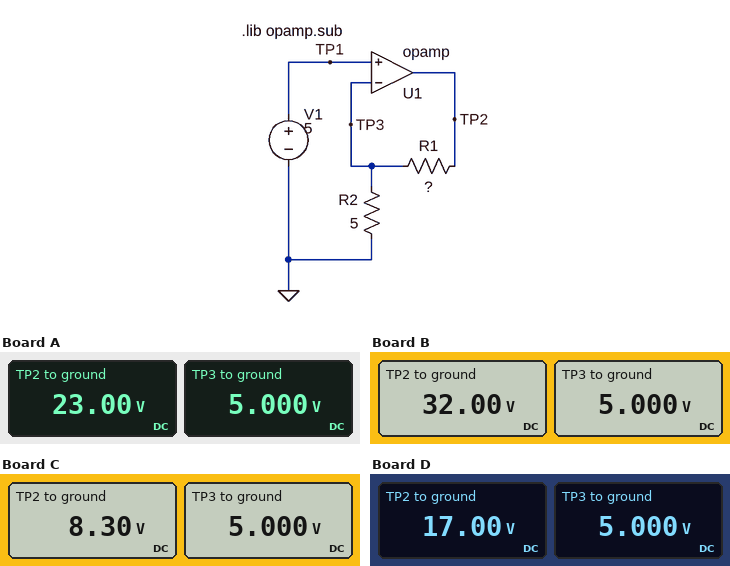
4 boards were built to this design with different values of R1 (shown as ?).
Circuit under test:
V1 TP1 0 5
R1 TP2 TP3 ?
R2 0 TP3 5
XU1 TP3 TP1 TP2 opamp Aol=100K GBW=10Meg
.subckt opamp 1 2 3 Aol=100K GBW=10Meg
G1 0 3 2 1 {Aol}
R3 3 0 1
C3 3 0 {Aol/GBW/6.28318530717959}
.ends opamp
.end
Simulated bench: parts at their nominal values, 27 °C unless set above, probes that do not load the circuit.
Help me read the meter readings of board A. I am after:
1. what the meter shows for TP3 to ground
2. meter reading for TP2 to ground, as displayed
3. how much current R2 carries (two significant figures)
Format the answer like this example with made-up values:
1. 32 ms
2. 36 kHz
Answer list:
1. 5.000 V
2. 23.00 V
3. 1.0 A
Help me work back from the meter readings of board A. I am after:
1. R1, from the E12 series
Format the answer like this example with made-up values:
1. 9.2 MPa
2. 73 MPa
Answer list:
1. 18 Ω
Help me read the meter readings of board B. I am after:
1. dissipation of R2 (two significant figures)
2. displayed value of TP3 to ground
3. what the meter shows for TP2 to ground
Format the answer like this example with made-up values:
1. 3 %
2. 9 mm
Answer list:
1. 5.0 W
2. 5.000 V
3. 32.00 V
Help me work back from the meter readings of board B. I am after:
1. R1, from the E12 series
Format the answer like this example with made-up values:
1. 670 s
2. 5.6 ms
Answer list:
1. 27 Ω
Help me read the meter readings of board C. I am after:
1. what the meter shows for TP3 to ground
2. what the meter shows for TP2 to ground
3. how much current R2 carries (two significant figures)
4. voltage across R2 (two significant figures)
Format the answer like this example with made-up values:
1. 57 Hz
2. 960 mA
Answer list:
1. 5.000 V
2. 8.30 V
3. 1.0 A
4. 5.0 V
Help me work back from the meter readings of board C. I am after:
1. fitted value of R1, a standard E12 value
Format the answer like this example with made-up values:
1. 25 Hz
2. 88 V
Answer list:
1. 3.3 Ω
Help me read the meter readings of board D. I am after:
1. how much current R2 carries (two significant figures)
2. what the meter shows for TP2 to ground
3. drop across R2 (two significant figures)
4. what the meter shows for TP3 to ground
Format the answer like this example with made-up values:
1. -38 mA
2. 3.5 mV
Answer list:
1. 1.0 A
2. 17.00 V
3. 5.0 V
4. 5.000 V
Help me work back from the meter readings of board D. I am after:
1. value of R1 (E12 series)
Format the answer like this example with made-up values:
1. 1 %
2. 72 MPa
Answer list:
1. 12 Ω
